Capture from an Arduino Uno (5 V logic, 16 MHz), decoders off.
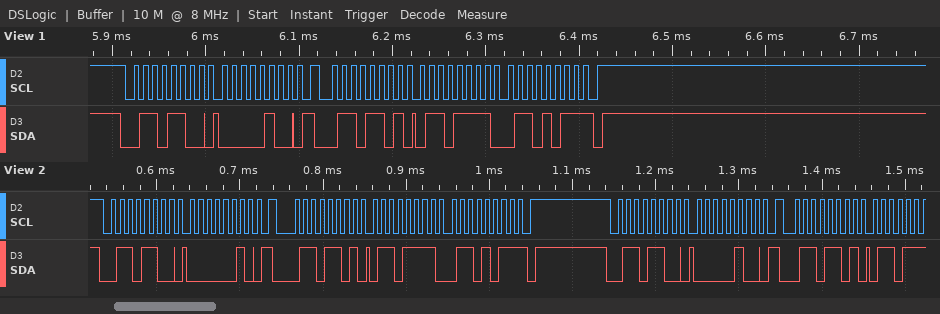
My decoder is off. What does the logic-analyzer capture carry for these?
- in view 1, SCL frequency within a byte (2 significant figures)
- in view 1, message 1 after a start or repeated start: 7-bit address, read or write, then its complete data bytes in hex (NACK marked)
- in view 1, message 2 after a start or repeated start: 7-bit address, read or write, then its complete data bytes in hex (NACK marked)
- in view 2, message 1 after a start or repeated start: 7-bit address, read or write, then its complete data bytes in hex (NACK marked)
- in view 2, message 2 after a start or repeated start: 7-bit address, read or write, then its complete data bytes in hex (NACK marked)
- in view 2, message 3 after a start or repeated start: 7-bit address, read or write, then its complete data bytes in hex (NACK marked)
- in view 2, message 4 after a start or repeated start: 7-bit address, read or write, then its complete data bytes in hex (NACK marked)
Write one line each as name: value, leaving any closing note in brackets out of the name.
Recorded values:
in view 1, SCL frequency within a byte: 100 kHz
in view 1, message 1 after a start or repeated start: 7-bit address, read or write, then its complete data bytes in hex: 0x36 write: 04
in view 1, message 2 after a start or repeated start: 7-bit address, read or write, then its complete data bytes in hex: 0x36 read: 6F 6B NACK
in view 2, message 1 after a start or repeated start: 7-bit address, read or write, then its complete data bytes in hex: 0x36 write: 02
in view 2, message 2 after a start or repeated start: 7-bit address, read or write, then its complete data bytes in hex: 0x36 read: 6F 6B NACK
in view 2, message 3 after a start or repeated start: 7-bit address, read or write, then its complete data bytes in hex: 0x36 write: 04
in view 2, message 4 after a start or repeated start: 7-bit address, read or write, then its complete data bytes in hex: 0x36 read
